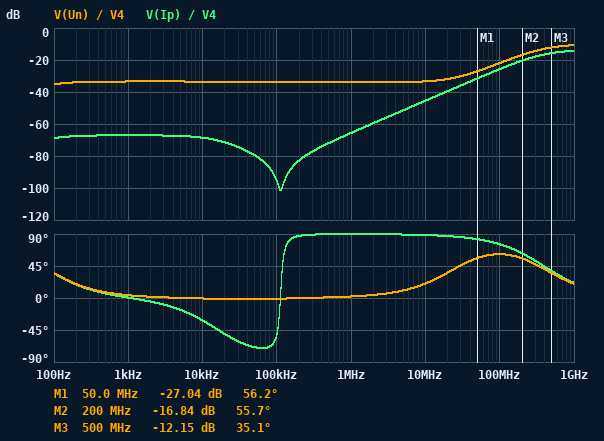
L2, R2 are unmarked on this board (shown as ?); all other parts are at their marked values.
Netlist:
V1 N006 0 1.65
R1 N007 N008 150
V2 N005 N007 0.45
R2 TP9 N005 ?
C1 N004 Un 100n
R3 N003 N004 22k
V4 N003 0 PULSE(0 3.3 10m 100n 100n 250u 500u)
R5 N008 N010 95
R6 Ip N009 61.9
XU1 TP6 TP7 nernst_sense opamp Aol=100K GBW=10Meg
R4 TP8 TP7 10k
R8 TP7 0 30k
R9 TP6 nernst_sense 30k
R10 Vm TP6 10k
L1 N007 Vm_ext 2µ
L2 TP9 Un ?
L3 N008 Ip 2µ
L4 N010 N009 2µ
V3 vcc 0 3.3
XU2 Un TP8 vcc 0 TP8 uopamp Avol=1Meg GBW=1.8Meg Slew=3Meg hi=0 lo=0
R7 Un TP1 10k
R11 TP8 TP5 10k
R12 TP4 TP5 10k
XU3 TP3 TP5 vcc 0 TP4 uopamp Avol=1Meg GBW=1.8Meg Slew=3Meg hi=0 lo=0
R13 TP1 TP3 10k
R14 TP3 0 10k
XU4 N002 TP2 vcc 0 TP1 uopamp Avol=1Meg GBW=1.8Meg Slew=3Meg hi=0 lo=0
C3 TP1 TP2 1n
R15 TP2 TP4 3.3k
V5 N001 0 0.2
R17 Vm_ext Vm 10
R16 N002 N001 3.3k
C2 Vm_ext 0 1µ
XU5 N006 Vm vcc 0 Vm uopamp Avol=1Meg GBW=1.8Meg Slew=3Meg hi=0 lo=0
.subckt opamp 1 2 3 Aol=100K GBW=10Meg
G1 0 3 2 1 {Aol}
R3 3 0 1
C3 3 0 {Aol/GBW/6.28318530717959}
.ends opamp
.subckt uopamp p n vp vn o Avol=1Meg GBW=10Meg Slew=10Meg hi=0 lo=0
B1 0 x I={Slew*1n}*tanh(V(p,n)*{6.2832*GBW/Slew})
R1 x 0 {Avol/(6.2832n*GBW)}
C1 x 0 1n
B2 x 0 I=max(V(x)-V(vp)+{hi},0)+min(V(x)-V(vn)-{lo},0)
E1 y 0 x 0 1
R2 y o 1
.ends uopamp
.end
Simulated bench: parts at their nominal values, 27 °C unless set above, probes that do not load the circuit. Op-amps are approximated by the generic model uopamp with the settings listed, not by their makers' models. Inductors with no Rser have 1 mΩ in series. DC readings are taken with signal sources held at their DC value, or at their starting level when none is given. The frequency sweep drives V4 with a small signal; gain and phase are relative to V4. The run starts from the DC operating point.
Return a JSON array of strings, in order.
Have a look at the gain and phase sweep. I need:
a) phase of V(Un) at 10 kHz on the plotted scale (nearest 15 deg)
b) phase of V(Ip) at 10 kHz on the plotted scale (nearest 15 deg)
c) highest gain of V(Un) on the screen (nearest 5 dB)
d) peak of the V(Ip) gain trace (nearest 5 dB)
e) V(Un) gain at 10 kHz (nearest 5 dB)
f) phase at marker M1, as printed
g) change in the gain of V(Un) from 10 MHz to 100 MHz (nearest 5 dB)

["0 deg", "-30 deg", "-10 dB", "-15 dB", "-35 dB", "56.2 deg", "10 dB"]
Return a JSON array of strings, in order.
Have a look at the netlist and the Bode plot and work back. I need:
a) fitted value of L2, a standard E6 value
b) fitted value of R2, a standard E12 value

["1 µH", "470 Ω"]
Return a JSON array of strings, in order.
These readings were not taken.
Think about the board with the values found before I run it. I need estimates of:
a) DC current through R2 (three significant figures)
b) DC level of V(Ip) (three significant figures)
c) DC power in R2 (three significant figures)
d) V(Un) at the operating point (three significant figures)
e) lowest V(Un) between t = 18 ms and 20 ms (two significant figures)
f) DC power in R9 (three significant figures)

["20.0 µA", "1.65 V", "188 nW", "2.11 V", "2.1 V", "1.38 µW"]
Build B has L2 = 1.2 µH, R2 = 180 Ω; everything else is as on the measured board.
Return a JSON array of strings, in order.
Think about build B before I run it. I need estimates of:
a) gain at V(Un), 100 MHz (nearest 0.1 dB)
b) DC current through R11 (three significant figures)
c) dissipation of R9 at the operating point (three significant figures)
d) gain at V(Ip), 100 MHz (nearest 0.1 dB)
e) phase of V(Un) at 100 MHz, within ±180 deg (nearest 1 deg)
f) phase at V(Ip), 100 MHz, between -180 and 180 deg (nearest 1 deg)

["-21.3 dB", "95.2 µA", "1.56 µW", "-25.4 dB", "69 deg", "74 deg"]
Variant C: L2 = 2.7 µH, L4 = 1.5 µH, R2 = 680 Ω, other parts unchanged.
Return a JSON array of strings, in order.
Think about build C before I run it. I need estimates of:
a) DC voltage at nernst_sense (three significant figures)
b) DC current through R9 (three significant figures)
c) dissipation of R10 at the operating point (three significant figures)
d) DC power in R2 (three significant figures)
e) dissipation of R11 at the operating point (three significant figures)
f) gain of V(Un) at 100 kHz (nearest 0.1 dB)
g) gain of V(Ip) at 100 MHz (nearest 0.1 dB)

["1.39 V", "6.47 µA", "418 nW", "272 nW", "91.6 µW", "-31.0 dB", "-26.3 dB"]
